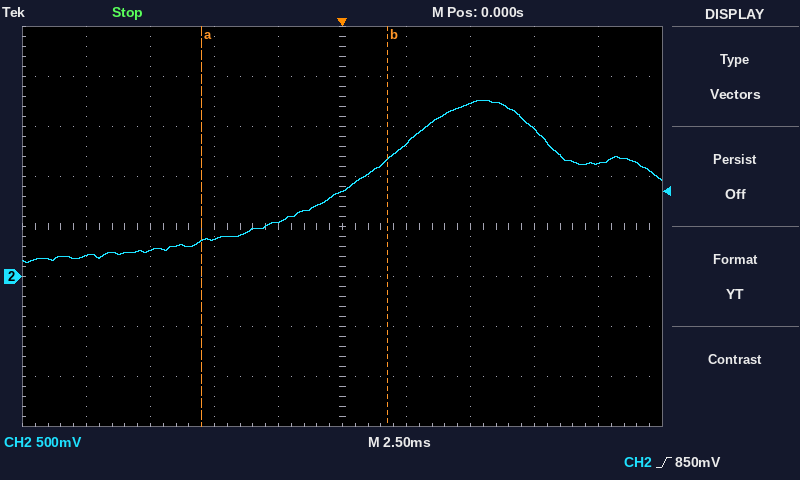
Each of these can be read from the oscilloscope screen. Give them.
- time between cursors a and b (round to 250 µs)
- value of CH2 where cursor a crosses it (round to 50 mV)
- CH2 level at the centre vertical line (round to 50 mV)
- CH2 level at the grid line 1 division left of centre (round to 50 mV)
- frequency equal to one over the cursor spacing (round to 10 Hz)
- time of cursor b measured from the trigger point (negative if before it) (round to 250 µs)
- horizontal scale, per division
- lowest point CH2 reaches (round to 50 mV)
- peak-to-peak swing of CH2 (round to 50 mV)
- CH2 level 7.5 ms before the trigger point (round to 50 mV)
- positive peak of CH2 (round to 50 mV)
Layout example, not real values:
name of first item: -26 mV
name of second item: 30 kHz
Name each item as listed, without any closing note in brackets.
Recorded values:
time between cursors a and b: 7.25 ms
value of CH2 where cursor a crosses it: 350 mV
CH2 level at the centre vertical line: 850 mV
CH2 level at the grid line 1 division left of centre: 550 mV
frequency equal to one over the cursor spacing: 140 Hz
time of cursor b measured from the trigger point (negative if before it): +1.75 ms
horizontal scale, per division: 2.5 ms
lowest point CH2 reaches: 150 mV
peak-to-peak swing of CH2: 1.60 V
CH2 level 7.5 ms before the trigger point: 250 mV
positive peak of CH2: 1.75 V
